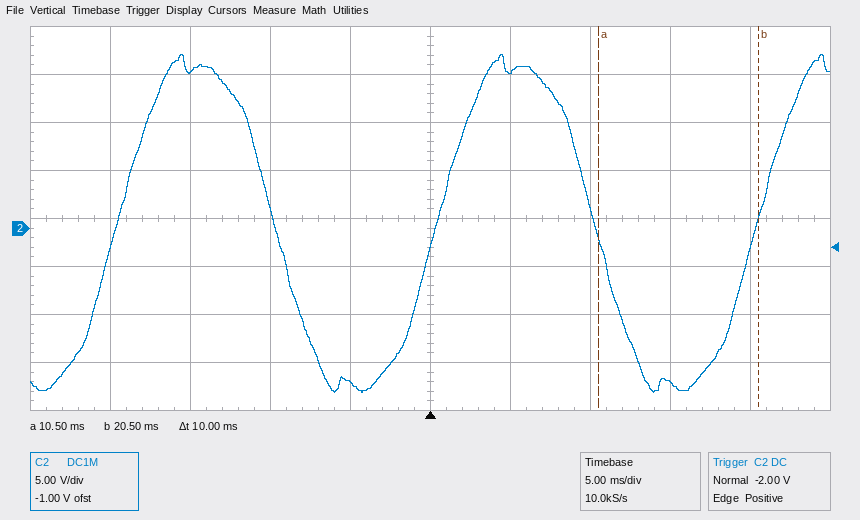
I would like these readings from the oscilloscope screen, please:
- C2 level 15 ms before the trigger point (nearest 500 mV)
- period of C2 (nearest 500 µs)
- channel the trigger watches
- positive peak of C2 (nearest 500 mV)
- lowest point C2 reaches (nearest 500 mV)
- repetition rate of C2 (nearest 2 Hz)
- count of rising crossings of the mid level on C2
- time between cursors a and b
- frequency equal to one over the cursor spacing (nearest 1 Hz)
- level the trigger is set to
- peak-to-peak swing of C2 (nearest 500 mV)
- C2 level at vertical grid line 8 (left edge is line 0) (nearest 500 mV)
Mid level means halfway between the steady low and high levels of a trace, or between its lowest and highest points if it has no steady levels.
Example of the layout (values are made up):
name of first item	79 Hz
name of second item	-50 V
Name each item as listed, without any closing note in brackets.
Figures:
C2 level 15 ms before the trigger point	16.5 V
period of C2	20.0 ms
channel the trigger watches	C2
positive peak of C2	18.0 V
lowest point C2 reaches	-17.0 V
repetition rate of C2	50 Hz
count of rising crossings of the mid level on C2	3
time between cursors a and b	10 ms
frequency equal to one over the cursor spacing	100 Hz
level the trigger is set to	-2.00 V
peak-to-peak swing of C2	35.0 V
C2 level at vertical grid line 8 (left edge is line 0)	-16.0 V
